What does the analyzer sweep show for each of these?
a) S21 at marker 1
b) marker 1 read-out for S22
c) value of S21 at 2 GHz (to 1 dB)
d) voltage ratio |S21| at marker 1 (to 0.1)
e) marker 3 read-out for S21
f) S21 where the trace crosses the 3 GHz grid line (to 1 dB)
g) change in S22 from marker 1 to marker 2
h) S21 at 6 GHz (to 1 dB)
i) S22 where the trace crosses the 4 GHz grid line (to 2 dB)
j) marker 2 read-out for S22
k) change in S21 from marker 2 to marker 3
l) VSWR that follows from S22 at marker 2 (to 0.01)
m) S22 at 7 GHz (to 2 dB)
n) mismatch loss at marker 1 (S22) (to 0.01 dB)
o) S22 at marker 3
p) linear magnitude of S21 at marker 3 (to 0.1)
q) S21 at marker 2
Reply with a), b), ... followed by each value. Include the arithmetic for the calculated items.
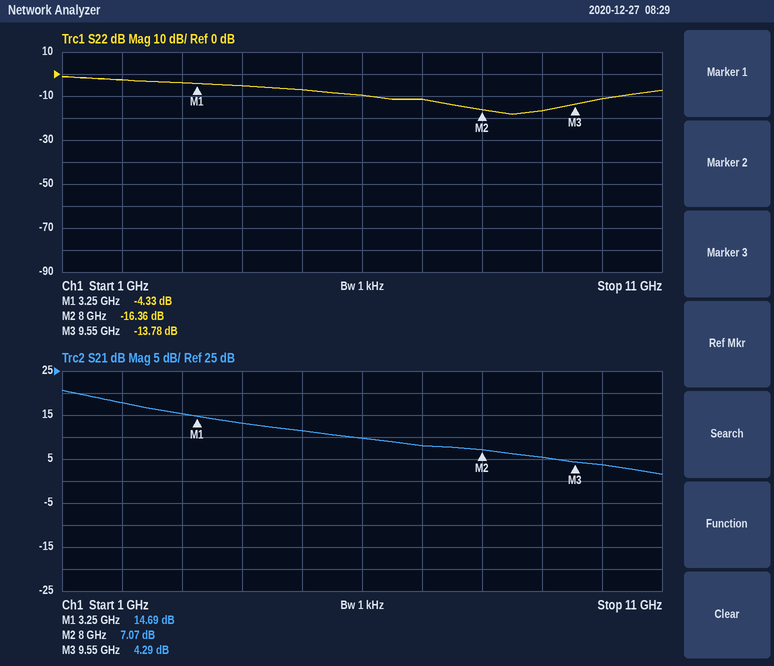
a) 14.69 dB
b) -4.33 dB
c) 18 dB
d) 10^(14.69/20) ≈ 5.4
e) 4.29 dB
f) 15 dB
g) -16.36 − (-4.33) = -12.03 dB
h) 10 dB
i) -6 dB
j) -16.36 dB
k) 4.29 − (7.07) = -2.78 dB
l) (1 + 0.1521)/(1 − 0.1521) ≈ 1.36
m) -12 dB
n) −10 log10(1 − 10^(-4.33/10)) ≈ 2.00 dB
o) -13.78 dB
p) 10^(4.29/20) ≈ 1.6
q) 7.07 dB
